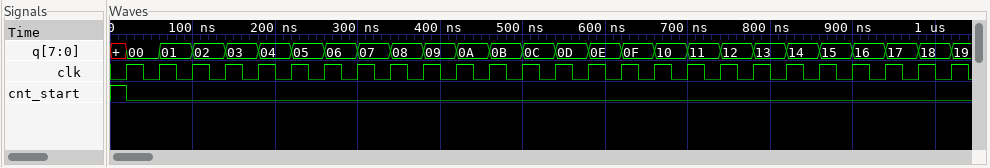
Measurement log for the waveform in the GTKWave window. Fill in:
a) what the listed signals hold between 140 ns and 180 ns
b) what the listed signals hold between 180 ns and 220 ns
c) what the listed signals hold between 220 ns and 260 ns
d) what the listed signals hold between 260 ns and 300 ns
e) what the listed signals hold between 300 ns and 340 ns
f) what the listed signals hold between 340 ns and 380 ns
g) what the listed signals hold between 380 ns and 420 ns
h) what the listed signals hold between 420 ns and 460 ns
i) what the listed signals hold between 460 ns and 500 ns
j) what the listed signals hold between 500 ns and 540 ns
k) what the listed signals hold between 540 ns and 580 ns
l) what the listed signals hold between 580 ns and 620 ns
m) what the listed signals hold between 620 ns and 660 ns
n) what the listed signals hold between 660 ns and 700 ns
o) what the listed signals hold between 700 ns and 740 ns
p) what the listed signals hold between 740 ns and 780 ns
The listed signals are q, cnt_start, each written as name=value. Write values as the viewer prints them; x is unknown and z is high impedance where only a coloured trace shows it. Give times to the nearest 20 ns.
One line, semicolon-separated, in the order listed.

q=03, cnt_start=0; q=04, cnt_start=0; q=05, cnt_start=0; q=06, cnt_start=0; q=07, cnt_start=0; q=08, cnt_start=0; q=09, cnt_start=0; q=0A, cnt_start=0; q=0B, cnt_start=0; q=0C, cnt_start=0; q=0D, cnt_start=0; q=0E, cnt_start=0; q=0F, cnt_start=0; q=10, cnt_start=0; q=11, cnt_start=0; q=12, cnt_start=0
